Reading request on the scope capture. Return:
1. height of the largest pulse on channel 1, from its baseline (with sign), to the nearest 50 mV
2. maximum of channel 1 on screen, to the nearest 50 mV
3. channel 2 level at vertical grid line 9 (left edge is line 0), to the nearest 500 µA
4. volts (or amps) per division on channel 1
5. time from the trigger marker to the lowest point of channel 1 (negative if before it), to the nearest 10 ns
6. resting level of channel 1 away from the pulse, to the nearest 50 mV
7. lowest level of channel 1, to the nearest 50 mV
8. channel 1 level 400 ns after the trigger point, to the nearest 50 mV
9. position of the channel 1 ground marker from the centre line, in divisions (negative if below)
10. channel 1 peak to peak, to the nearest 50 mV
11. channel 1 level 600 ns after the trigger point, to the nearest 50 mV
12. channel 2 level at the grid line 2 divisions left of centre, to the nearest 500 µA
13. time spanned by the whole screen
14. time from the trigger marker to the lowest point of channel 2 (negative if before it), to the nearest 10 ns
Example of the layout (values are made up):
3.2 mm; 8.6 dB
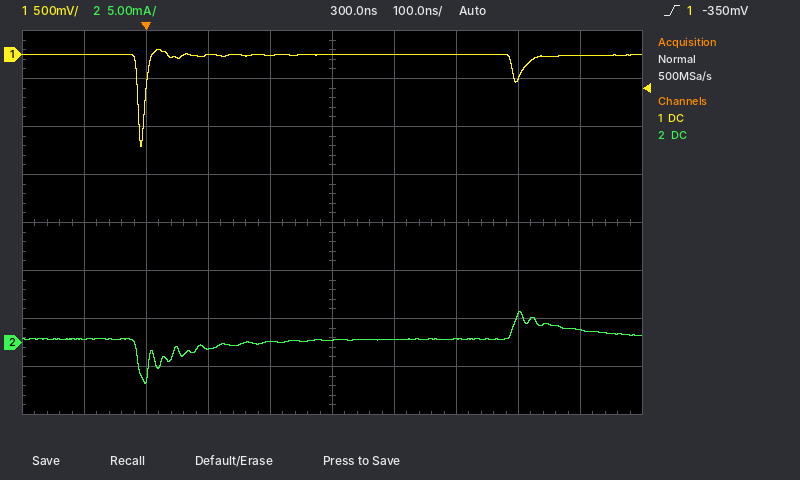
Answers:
-950 mV; 50 mV; 1.5 mA; 500 mV; -10 ns; 0 mV; -950 mV; 0 mV; +3.5 div; 1.00 V; -250 mV; -500 µA; 1 µs; 0 ns
